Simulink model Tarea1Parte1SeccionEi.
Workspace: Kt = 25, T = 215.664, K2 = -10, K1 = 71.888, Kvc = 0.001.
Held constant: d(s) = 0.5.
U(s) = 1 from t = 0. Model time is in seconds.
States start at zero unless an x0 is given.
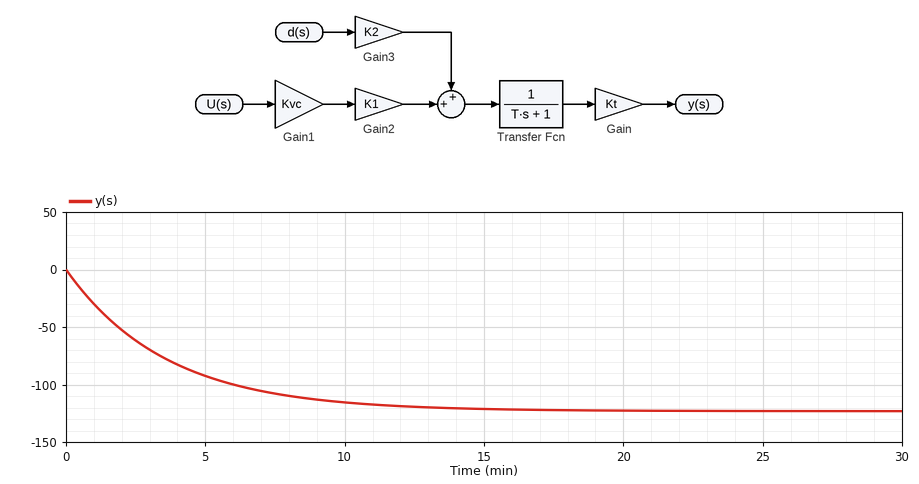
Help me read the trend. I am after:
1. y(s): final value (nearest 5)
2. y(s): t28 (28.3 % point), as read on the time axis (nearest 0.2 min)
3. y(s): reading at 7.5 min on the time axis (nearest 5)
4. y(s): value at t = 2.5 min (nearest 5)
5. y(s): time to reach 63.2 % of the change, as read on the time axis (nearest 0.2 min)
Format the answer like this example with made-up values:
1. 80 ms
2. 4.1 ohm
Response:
1. -125
2. 1.2 min
3. -110
4. -60
5. 3.6 min
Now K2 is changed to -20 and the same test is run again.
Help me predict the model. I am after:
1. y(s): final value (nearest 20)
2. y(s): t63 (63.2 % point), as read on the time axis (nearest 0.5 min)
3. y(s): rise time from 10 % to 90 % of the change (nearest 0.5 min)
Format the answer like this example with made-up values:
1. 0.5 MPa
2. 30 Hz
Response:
1. -240
2. 3.5 min
3. 8.0 min
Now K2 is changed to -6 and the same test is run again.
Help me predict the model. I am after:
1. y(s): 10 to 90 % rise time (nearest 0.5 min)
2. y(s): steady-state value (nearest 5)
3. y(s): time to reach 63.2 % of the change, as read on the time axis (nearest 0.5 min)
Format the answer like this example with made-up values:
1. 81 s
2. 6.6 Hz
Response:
1. 8.0 min
2. -75
3. 3.5 min
